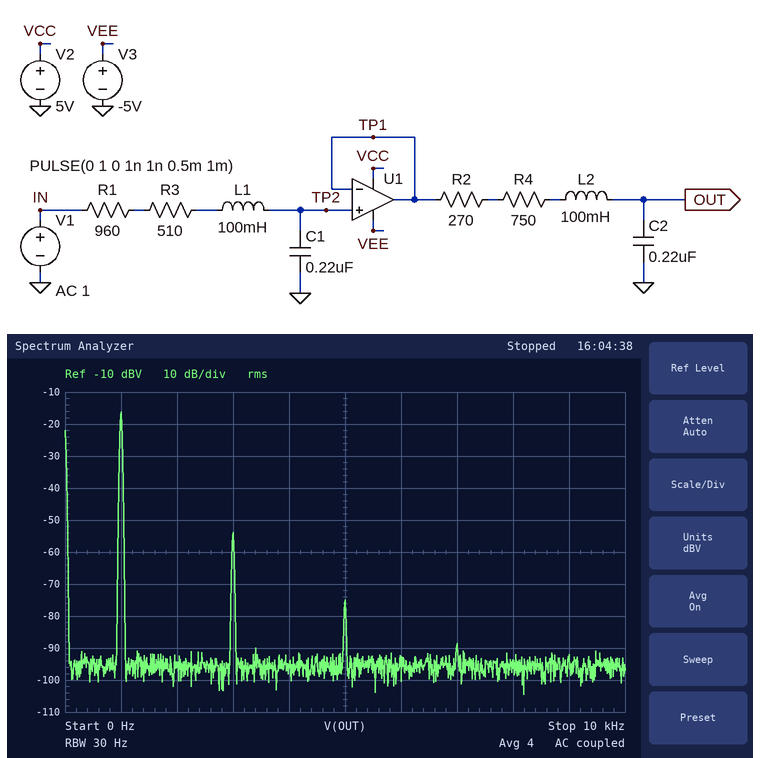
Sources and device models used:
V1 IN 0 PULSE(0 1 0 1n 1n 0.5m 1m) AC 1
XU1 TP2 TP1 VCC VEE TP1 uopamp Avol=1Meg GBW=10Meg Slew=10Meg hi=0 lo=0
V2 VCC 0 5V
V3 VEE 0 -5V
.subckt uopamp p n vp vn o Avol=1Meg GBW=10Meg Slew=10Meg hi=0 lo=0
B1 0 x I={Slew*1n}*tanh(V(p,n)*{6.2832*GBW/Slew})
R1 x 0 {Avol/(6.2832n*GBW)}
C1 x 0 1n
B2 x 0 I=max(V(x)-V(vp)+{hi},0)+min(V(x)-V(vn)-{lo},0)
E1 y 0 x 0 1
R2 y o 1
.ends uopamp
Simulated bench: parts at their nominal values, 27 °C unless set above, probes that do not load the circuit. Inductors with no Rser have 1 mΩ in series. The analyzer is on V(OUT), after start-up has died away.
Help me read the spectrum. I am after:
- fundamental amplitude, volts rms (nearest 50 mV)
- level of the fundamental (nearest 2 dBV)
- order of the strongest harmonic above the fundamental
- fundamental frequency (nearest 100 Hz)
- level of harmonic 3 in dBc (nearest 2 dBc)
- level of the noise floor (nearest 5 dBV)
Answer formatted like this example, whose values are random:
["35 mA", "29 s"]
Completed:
["150 mV", "-16 dBV", "3", "1.0 kHz", "-38 dBc", "-95 dBV"]
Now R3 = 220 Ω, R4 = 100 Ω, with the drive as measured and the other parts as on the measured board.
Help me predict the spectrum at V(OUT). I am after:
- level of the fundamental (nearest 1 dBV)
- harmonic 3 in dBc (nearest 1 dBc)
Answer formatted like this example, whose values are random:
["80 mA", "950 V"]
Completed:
["-6 dBV", "-46 dBc"]
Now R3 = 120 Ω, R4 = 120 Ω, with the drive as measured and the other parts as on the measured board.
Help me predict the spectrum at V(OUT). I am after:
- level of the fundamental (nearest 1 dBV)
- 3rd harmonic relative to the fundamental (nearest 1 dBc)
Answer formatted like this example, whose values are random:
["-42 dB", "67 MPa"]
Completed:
["-5 dBV", "-46 dBc"]
